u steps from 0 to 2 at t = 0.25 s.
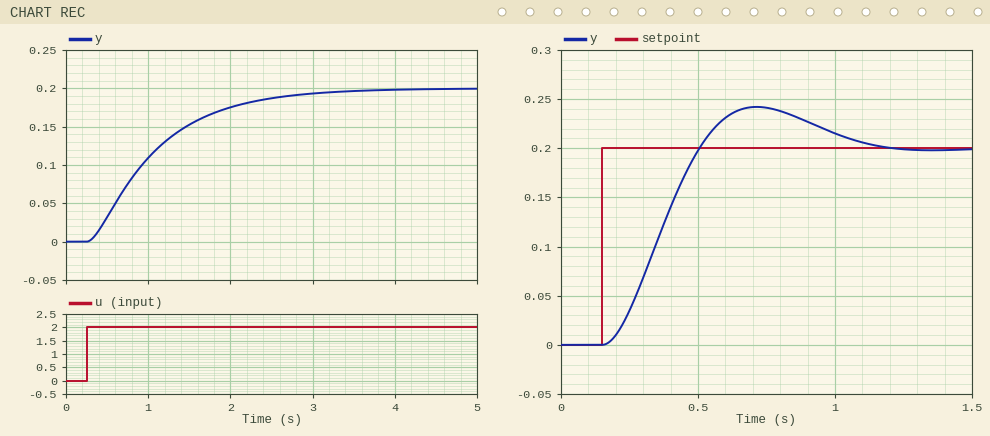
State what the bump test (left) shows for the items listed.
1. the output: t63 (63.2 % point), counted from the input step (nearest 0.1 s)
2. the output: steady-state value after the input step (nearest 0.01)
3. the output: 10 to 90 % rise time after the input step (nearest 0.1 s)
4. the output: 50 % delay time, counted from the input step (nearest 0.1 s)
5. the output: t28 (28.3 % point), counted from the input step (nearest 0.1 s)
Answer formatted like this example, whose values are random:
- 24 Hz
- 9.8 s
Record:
- 0.9 s
- 0.20
- 1.7 s
- 0.7 s
- 0.4 s
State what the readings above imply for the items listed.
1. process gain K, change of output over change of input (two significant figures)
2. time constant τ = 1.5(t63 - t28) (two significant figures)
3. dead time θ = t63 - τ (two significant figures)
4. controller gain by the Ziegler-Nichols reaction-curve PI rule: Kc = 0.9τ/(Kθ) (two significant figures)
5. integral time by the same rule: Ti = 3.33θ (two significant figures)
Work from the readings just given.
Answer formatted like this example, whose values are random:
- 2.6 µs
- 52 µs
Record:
- 0.10
- 0.75 s
- 0.15 s
- 45
- 0.50 s
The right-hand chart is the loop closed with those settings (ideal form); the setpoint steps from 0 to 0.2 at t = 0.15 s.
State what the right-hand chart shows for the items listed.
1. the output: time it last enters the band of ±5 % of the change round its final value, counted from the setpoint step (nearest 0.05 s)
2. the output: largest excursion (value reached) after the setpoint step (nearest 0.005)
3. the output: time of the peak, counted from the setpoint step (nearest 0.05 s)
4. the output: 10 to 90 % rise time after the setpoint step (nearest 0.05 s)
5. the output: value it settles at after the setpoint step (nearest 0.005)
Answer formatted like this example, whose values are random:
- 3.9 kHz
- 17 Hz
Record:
- 0.90 s
- 0.240
- 0.55 s
- 0.25 s
- 0.200
